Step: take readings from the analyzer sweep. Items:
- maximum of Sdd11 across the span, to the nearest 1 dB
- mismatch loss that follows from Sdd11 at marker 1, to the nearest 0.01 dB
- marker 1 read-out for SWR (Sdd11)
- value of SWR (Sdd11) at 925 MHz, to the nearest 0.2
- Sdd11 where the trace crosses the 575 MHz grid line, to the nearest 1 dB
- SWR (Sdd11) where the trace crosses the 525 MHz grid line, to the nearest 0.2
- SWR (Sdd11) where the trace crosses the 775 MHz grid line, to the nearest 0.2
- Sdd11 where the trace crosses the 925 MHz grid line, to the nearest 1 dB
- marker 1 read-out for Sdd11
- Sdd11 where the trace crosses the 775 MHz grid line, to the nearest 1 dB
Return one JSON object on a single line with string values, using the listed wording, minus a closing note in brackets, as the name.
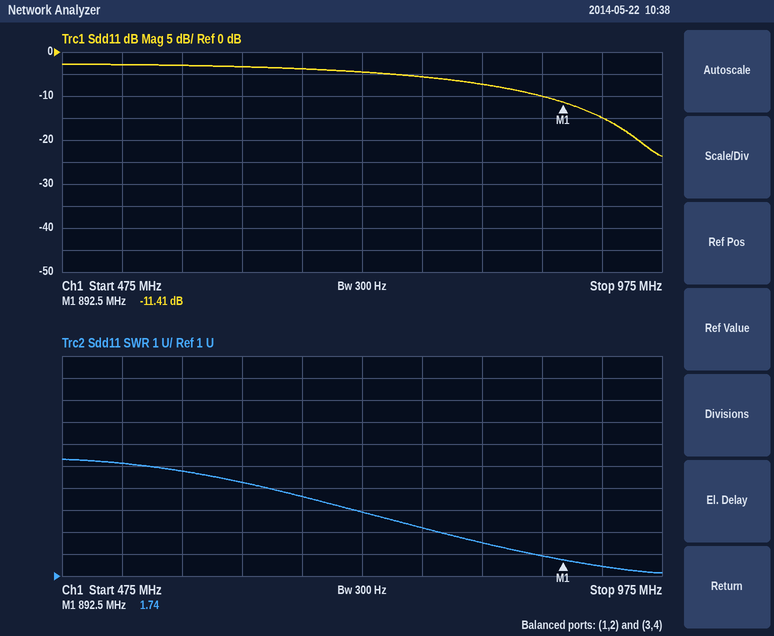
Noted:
{"maximum of Sdd11 across the span, to the nearest 1 dB": "-3 dB", "mismatch loss that follows from Sdd11 at marker 1, to the nearest 0.01 dB": "0.33 dB", "marker 1 read-out for SWR": "1.74", "value of SWR (Sdd11) at 925 MHz, to the nearest 0.2": "1.4", "Sdd11 where the trace crosses the 575 MHz grid line, to the nearest 1 dB": "-3 dB", "SWR (Sdd11) where the trace crosses the 525 MHz grid line, to the nearest 0.2": "6.2", "SWR (Sdd11) where the trace crosses the 775 MHz grid line, to the nearest 0.2": "3.2", "Sdd11 where the trace crosses the 925 MHz grid line, to the nearest 1 dB": "-15 dB", "marker 1 read-out for Sdd11": "-11.41 dB", "Sdd11 where the trace crosses the 775 MHz grid line, to the nearest 1 dB": "-6 dB"}
